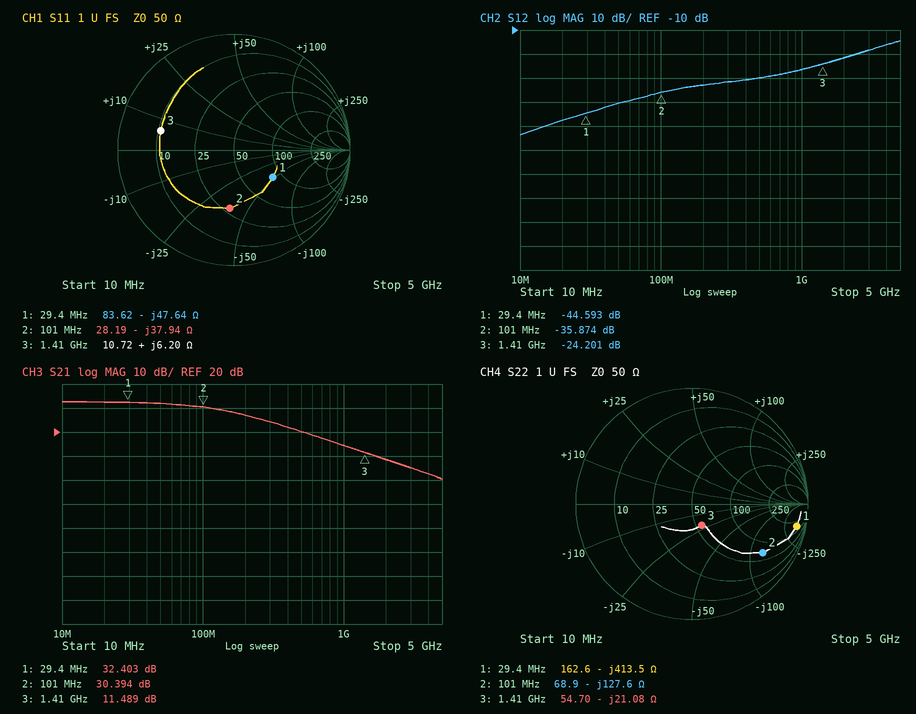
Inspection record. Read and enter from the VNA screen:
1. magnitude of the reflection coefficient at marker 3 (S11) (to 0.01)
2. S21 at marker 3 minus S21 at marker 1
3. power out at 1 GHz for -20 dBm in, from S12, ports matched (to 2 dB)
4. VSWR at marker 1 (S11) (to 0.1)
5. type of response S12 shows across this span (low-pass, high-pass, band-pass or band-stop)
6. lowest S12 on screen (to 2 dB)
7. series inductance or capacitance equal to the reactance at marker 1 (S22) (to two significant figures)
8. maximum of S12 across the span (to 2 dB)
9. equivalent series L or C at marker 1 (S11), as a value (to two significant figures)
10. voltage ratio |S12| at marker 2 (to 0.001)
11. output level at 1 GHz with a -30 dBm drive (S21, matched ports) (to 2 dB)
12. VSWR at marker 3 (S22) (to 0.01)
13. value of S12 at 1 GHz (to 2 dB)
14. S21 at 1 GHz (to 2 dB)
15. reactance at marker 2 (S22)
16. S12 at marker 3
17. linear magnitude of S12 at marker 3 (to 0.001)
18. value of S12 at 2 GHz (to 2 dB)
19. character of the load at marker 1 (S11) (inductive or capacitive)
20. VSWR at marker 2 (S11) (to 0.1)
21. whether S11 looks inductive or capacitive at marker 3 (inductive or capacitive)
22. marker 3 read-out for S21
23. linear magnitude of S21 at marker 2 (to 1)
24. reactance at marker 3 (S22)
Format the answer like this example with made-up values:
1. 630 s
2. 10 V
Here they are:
1. 0.65
2. -20.914 dB
3. -46 dBm
4. 2.4
5. high-pass
6. -54 dB
7. 13 pF
8. -14 dB
9. 110 pF
10. 0.016
11. -16 dBm
12. 1.51
13. -26 dB
14. 14 dB
15. -127.6 Ω
16. -24.201 dB
17. 0.062
18. -22 dB
19. capacitive
20. 3.0
21. inductive
22. 11.489 dB
23. 33
24. -21.08 Ω
